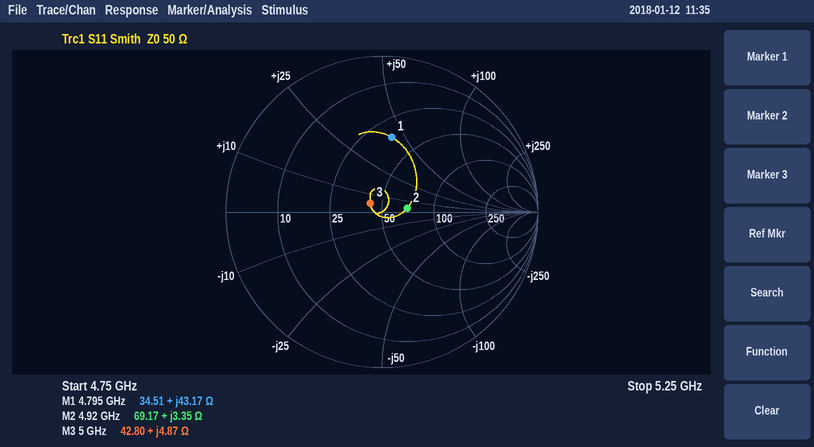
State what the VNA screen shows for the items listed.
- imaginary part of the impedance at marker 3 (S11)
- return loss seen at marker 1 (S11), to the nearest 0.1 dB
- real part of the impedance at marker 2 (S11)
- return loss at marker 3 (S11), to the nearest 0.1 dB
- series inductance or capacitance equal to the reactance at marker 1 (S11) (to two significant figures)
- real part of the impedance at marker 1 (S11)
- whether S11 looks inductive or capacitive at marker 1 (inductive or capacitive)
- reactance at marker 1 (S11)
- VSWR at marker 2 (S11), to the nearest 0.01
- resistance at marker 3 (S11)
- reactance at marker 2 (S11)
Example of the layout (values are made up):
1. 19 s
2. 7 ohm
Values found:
1. +4.87 Ω
2. 6.3 dB
3. 69.17 Ω
4. 20.6 dB
5. 1.4 nH
6. 34.51 Ω
7. inductive
8. +43.17 Ω
9. 1.39
10. 42.80 Ω
11. +3.35 Ω
